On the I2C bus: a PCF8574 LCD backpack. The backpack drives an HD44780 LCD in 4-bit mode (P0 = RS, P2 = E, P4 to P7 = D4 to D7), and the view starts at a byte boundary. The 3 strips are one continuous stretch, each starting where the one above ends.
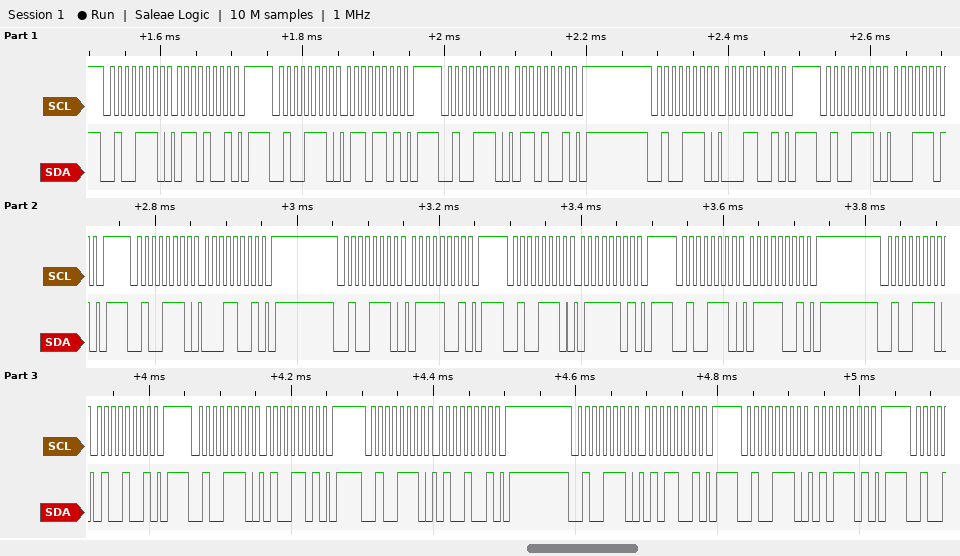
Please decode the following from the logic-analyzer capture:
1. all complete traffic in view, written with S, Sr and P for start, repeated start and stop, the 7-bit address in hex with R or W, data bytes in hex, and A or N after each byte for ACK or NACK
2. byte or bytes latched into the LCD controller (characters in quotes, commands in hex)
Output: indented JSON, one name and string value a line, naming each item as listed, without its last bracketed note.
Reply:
{
  "all complete traffic in view, written with S, Sr and P for start, repeated start and stop, the 7-bit address in hex with R or W, data bytes in hex, and A or N after each byte for ACK or NACK": "S 27W A 69 A P S 27W A 6D A P S 27W A 69 A P S 27W A 19 A P S 27W A 1D A P S 27W A 19 A P S 27W A 79 A P S 27W A 7D A P S 27W A 79 A P S 27W A 49 A P S 27W A 4D A P S 27W A 49 A P S 27W A 59 A P S 27W A 5D A P",
  "byte or bytes latched into the LCD controller": "'a' 't'"
}
